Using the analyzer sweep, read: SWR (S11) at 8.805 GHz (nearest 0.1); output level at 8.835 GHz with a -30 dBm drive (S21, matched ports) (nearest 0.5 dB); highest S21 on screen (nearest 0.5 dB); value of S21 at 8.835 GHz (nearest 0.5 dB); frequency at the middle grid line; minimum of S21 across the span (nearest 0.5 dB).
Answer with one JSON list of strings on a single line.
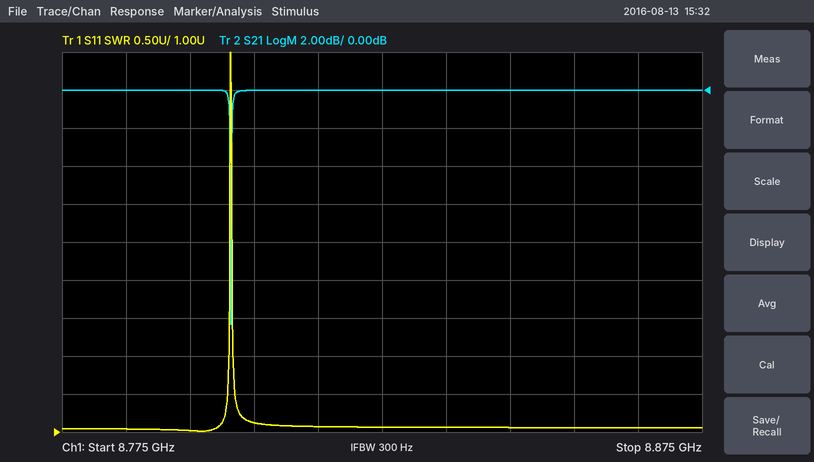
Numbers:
["1.1", "-30.0 dBm", "0.0 dB", "0.0 dB", "8.825 GHz", "-12.5 dB"]
